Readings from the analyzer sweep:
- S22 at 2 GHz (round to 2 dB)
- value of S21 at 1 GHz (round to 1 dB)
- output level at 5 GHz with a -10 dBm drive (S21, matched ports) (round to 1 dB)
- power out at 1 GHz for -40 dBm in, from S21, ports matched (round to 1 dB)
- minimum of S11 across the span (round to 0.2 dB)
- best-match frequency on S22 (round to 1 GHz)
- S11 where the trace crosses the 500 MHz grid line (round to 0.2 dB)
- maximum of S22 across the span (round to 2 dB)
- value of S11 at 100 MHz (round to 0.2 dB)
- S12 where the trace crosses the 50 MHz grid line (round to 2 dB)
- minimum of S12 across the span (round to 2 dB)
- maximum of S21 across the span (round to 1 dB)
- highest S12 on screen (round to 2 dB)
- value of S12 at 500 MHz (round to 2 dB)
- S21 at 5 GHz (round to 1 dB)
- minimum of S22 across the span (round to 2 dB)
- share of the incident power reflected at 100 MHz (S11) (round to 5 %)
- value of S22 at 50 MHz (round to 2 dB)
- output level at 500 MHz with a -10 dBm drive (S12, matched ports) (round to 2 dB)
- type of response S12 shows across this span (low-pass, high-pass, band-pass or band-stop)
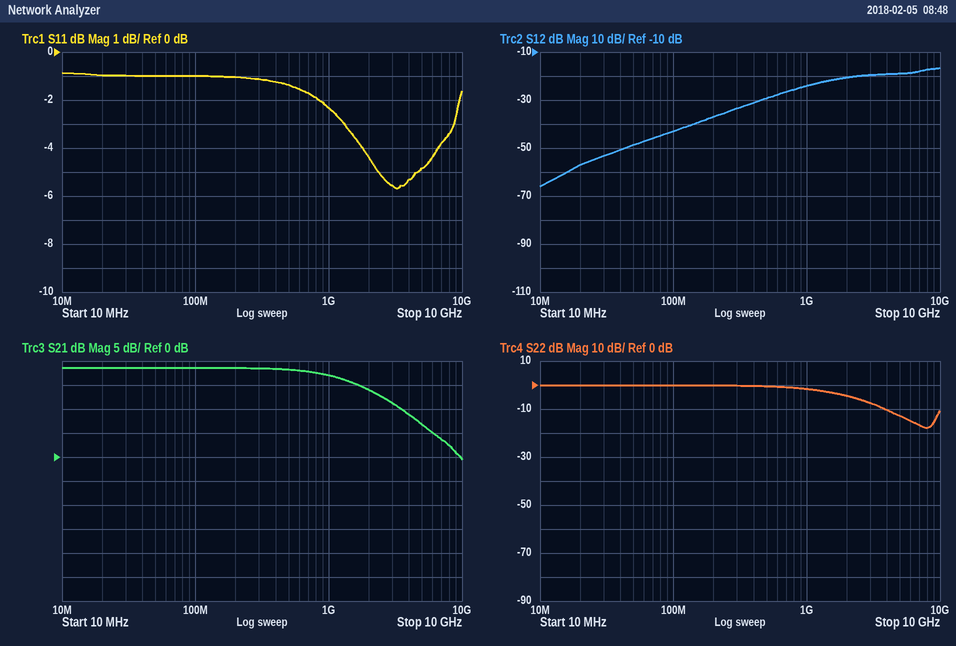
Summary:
-4 dB
17 dB
-3 dBm
-23 dBm
-5.6 dB
8 GHz
-1.4 dB
0 dB
-1.0 dB
-48 dB
-66 dB
19 dB
-16 dB
-30 dB
7 dB
-18 dB
80 %
0 dB
-40 dBm
high-pass
